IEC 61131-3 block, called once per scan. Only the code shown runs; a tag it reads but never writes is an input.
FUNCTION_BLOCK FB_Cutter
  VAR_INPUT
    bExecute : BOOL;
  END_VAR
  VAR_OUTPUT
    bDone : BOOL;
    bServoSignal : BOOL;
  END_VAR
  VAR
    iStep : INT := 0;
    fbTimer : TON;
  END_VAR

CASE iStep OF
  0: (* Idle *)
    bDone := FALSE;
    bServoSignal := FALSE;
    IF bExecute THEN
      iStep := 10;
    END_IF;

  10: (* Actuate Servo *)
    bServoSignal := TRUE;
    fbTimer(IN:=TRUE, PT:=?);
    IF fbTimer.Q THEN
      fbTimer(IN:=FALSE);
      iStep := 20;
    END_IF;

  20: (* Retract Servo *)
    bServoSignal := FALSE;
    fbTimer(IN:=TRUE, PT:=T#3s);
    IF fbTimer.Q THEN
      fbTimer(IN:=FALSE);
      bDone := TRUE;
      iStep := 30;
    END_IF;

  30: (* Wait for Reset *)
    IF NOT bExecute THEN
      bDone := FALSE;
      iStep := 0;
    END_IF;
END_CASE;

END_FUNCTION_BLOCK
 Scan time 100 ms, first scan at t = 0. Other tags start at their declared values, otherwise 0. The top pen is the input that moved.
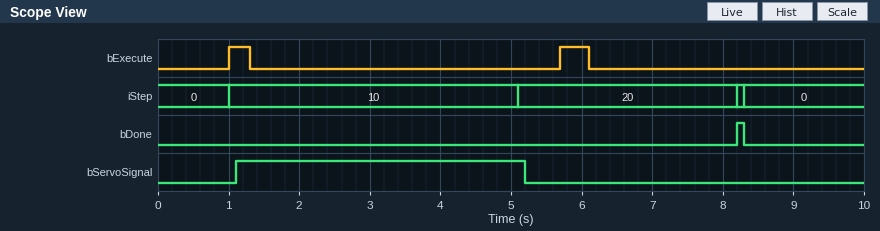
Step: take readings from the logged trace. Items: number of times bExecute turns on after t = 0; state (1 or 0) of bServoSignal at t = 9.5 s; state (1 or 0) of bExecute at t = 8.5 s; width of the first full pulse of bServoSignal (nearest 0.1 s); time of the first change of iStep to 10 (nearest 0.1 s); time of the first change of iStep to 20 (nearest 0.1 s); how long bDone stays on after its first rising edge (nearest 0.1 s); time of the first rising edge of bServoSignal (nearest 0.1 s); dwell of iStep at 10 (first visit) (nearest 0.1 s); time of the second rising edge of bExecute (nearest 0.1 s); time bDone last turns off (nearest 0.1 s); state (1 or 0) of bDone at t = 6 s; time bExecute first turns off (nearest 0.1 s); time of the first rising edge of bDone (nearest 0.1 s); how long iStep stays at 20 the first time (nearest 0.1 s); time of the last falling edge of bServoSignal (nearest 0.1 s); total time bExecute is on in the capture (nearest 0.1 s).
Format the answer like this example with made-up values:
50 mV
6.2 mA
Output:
2
0
0
4.1 s
1.0 s
5.1 s
0.1 s
1.1 s
4.1 s
5.7 s
8.3 s
0
1.3 s
8.2 s
3.1 s
5.2 s
0.7 s
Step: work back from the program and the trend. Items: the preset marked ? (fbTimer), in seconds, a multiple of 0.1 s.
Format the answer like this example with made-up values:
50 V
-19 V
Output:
4.0 s
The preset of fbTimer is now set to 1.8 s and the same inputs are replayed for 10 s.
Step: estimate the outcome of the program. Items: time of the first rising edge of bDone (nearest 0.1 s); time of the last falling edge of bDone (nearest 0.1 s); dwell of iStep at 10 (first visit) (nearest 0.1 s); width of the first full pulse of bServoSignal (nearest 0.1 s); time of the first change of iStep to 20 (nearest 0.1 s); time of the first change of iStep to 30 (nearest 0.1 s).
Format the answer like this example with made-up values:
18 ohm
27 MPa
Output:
6.0 s
6.1 s
1.9 s
1.9 s
2.9 s
6.0 s
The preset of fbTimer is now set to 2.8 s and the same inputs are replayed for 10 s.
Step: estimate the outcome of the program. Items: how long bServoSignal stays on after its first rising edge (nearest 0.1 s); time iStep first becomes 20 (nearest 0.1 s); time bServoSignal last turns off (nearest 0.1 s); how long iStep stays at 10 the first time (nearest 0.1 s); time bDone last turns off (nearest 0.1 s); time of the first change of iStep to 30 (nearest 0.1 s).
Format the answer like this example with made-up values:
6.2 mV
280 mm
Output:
2.9 s
3.9 s
4.0 s
2.9 s
7.1 s
7.0 s
